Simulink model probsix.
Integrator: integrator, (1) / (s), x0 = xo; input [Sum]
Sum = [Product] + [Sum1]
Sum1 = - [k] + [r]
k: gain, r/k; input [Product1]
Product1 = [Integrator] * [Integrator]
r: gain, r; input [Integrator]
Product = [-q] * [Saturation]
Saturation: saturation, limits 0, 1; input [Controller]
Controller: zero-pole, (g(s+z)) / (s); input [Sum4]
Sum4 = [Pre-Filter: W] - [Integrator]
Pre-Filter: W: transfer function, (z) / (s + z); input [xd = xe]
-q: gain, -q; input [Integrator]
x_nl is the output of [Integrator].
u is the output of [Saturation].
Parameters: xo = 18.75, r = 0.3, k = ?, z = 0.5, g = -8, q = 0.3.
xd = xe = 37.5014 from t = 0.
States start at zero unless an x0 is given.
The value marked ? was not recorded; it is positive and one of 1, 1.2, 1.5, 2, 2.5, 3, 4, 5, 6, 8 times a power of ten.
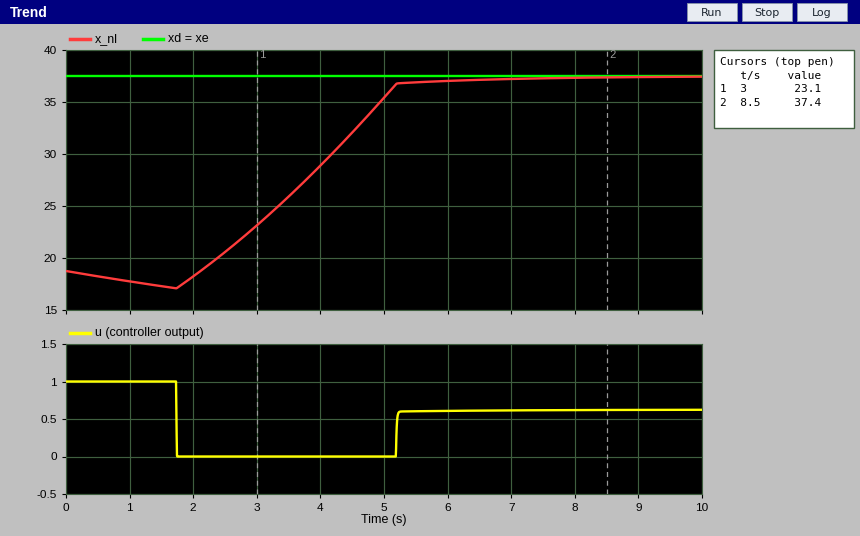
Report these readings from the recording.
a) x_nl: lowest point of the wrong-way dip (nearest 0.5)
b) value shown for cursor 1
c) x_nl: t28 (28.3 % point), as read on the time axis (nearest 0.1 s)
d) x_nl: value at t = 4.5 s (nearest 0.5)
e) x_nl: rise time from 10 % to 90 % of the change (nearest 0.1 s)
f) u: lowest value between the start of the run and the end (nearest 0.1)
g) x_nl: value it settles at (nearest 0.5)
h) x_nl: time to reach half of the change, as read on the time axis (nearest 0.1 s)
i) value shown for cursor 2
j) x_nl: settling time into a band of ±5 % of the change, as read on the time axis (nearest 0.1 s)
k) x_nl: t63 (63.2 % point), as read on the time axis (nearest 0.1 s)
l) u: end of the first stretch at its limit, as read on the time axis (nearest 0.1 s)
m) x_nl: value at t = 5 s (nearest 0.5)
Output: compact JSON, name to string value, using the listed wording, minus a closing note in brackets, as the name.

{"x_nl: lowest point of the wrong-way dip": "17.0", "value shown for cursor 1": "23.1", "x_nl: t28 (28.3 % point), as read on the time axis": "3.2 s", "x_nl: value at t = 4.5 s": "32.0", "x_nl: rise time from 10 % to 90 % of the change": "2.5 s", "u: lowest value between the start of the run and the end": "0.0", "x_nl: value it settles at": "37.5", "x_nl: time to reach half of the change, as read on the time axis": "3.9 s", "value shown for cursor 2": "37.4", "x_nl: settling time into a band of ±5 % of the change, as read on the time axis": "5.2 s", "x_nl: t63 (63.2 % point), as read on the time axis": "4.3 s", "u: end of the first stretch at its limit, as read on the time axis": "1.7 s", "x_nl: value at t = 5 s": "35.5"}
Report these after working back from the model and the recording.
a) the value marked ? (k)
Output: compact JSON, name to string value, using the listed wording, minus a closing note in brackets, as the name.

{"the value marked ?": "100"}
